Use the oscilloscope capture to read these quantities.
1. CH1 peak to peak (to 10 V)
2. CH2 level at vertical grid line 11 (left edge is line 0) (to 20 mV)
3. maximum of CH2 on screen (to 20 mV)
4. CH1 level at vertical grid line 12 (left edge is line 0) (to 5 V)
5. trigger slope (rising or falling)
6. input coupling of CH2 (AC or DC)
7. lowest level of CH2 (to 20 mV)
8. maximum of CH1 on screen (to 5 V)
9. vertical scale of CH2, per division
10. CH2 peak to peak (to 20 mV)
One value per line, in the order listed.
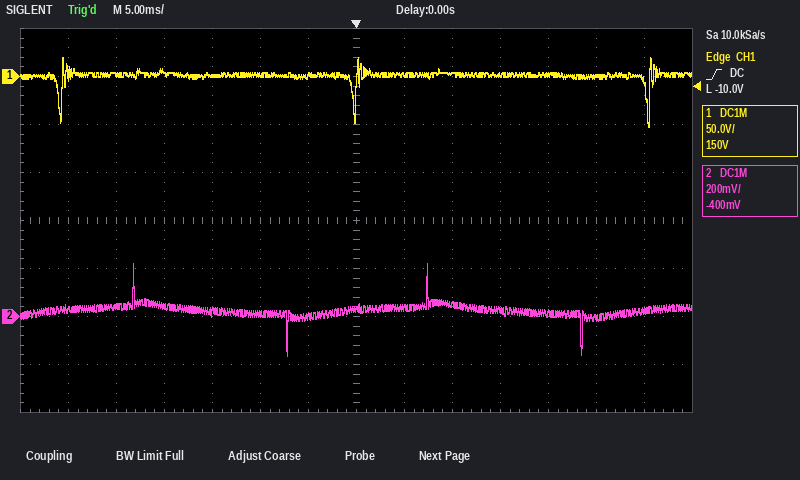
70 V
20 mV
220 mV
0 V
rising
DC
-160 mV
20 V
200 mV
380 mV
